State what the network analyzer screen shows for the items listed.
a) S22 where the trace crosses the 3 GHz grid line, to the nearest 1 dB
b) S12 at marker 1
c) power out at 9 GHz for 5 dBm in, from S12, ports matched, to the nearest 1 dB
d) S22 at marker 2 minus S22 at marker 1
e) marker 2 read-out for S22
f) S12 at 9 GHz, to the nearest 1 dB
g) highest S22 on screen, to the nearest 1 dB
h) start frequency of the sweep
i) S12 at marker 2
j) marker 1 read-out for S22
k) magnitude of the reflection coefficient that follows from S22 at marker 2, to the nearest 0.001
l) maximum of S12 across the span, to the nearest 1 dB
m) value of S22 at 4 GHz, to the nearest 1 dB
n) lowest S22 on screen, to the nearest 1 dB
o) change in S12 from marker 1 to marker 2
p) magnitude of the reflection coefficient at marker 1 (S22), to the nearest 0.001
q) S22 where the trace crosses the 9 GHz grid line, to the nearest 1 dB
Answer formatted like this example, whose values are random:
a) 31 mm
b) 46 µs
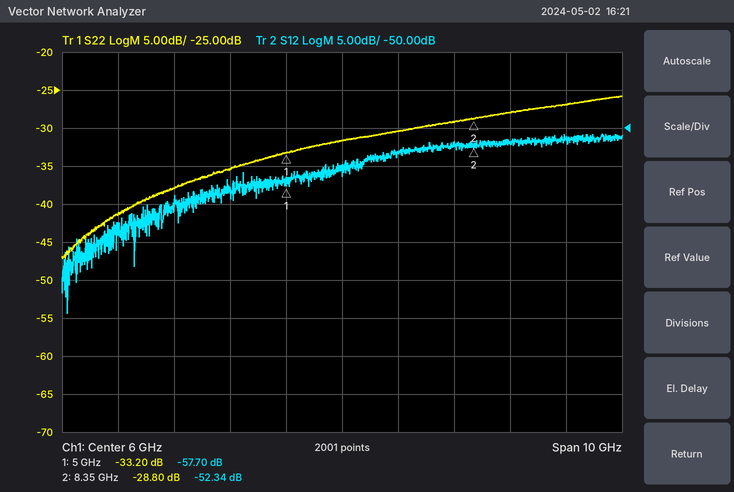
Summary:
a) -38 dB
b) -57.70 dB
c) -47 dBm
d) 4.40 dB
e) -28.80 dB
f) -52 dB
g) -26 dB
h) 1 GHz
i) -52.34 dB
j) -33.20 dB
k) 0.036
l) -51 dB
m) -35 dB
n) -47 dB
o) 5.36 dB
p) 0.022
q) -28 dB
